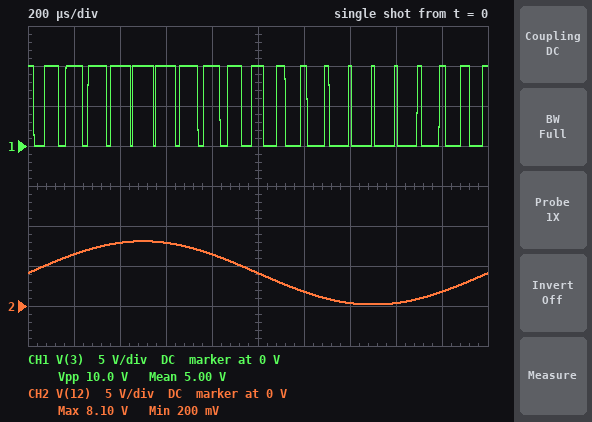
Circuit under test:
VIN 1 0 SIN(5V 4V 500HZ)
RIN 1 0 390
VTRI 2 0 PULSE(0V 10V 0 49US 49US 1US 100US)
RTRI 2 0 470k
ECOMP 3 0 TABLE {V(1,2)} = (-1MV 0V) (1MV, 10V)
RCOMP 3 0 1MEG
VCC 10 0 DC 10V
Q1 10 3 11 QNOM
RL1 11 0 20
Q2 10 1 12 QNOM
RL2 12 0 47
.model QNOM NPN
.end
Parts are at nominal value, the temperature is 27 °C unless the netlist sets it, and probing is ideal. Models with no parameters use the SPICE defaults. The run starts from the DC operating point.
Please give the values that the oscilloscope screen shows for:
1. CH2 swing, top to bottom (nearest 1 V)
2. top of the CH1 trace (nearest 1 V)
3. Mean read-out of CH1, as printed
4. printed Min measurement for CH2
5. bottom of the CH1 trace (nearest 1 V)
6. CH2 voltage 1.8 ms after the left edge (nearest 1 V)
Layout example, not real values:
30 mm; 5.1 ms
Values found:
8 V; 10 V; 5.00 V; 200 mV; 0 V; 2 V
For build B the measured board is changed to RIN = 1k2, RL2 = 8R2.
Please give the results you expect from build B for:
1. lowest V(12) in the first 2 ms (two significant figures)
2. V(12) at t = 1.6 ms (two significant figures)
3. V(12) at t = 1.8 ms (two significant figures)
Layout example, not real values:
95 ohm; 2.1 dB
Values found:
150 mV; 330 mV; 1.7 V
